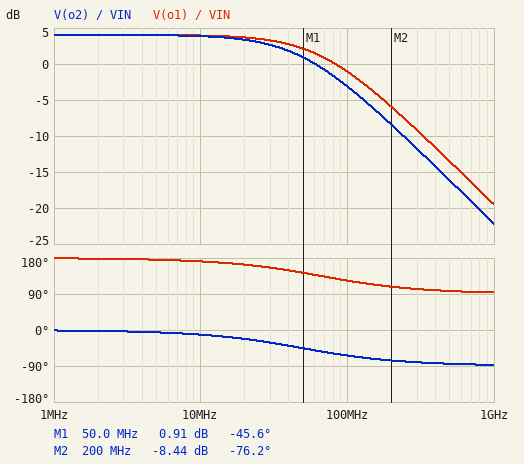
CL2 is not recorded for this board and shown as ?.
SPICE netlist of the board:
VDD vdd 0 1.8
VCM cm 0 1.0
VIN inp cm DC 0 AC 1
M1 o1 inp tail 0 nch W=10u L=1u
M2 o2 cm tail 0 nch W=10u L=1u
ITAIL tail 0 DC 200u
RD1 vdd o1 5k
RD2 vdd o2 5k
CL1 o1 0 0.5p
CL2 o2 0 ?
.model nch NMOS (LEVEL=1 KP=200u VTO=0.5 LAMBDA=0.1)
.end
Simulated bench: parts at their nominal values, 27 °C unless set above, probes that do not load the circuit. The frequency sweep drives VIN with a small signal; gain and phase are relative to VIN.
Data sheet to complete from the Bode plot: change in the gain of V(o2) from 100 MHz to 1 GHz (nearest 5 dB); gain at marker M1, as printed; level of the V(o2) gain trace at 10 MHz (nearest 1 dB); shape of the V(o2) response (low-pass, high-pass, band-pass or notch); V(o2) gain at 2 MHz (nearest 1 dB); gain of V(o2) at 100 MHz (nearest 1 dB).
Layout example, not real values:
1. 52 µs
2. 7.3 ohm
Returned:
1. -20 dB
2. 0.91 dB
3. 4 dB
4. low-pass
5. 4 dB
6. -3 dB
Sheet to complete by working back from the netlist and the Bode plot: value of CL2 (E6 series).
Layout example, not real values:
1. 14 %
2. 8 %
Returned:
1. 680 fF
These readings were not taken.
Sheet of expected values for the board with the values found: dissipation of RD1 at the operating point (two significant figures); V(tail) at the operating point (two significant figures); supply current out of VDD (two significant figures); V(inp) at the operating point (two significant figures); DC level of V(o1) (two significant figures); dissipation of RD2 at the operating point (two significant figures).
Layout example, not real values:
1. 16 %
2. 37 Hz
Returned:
1. 50 µW
2. 200 mV
3. 200 µA
4. 1.0 V
5. 1.3 V
6. 50 µW
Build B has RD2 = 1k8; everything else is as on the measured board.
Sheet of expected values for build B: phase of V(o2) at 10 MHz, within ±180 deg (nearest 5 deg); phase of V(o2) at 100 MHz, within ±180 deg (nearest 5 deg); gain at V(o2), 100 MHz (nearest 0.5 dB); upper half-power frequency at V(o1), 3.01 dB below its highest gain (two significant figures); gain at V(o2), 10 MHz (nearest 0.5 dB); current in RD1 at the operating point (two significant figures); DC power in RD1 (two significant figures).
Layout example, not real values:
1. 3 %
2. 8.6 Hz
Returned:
1. -5 deg
2. -35 deg
3. -6.5 dB
4. 65 MHz
5. -4.5 dB
6. 99 µA
7. 49 µW
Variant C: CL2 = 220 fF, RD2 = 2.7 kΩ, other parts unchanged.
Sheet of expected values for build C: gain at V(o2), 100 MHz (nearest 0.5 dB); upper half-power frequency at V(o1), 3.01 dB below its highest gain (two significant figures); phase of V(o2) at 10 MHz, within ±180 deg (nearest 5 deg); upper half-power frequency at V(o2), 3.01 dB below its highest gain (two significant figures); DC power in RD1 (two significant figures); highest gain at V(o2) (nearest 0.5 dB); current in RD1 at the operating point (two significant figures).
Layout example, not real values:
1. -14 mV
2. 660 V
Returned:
1. -1.5 dB
2. 65 MHz
3. 0 deg
4. 280 MHz
5. 49 µW
6. -1.0 dB
7. 99 µA
